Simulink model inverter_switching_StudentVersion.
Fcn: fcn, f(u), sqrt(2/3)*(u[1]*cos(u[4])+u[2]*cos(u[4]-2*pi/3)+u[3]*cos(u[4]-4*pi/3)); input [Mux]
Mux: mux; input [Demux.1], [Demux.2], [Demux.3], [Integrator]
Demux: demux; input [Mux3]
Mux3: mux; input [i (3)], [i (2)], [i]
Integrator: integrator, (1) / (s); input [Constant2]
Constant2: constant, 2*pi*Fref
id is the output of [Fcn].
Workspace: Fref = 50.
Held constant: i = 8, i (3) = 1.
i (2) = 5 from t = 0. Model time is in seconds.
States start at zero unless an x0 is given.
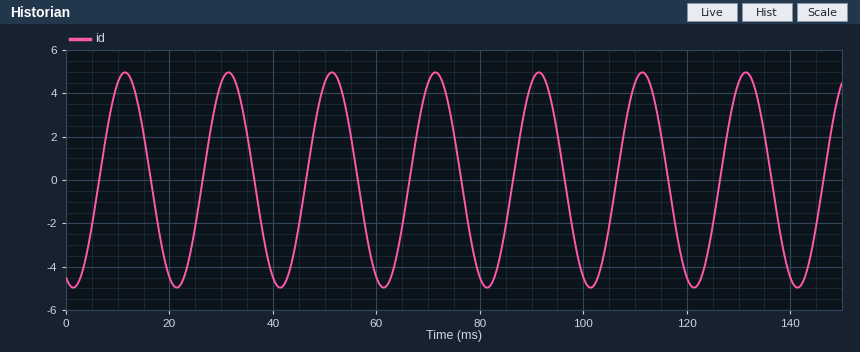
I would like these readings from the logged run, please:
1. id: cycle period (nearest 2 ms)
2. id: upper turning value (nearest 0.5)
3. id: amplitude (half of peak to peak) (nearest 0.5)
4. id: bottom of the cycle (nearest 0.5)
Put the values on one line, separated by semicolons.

20 ms; 5.0; 5.0; -5.0
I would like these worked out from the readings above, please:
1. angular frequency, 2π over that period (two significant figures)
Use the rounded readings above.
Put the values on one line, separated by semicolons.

0.31 rad/ms
